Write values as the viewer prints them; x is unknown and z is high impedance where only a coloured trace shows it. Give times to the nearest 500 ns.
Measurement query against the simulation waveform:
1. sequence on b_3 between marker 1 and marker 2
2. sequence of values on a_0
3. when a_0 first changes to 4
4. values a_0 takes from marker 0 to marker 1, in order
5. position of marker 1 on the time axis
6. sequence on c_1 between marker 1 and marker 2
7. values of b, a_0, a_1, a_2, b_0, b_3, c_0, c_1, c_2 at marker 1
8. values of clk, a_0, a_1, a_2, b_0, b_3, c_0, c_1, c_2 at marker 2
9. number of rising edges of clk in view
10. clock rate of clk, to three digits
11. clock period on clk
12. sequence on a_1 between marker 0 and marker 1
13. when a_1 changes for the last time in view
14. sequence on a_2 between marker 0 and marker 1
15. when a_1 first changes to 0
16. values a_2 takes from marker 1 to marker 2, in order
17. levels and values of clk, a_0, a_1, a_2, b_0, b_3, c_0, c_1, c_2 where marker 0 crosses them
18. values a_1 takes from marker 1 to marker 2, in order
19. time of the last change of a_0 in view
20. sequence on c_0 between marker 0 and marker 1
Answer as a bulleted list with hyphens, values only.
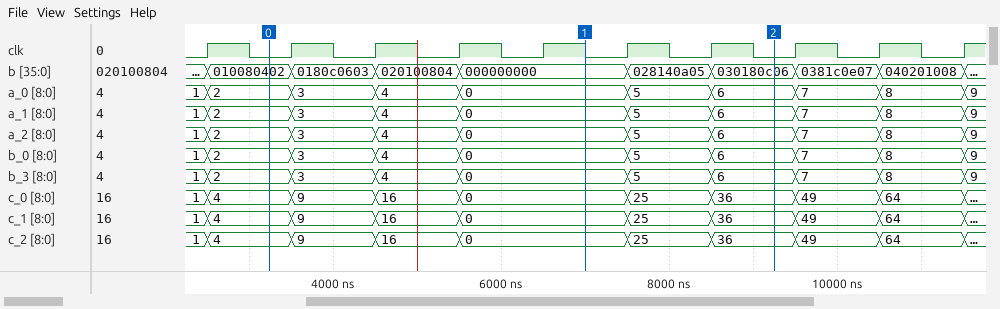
- 0, 5, 6
- 1, 2, 3, 4, 0, 5, 6, 7, 8, 9
- 4500 ns
- 2, 3, 4, 0
- 7000 ns
- 0, 25, 36
- b=000000000, a_0=0, a_1=0, a_2=0, b_0=0, b_3=0, c_0=0, c_1=0, c_2=0
- clk=0, a_0=6, a_1=6, a_2=6, b_0=6, b_3=6, c_0=36, c_1=36, c_2=36
- 10
- 1.00 MHz
- 1000 ns
- 2, 3, 4, 0
- 11500 ns
- 2, 3, 4, 0
- 5500 ns
- 0, 5, 6
- clk=0, a_0=2, a_1=2, a_2=2, b_0=2, b_3=2, c_0=4, c_1=4, c_2=4
- 0, 5, 6
- 11500 ns
- 4, 9, 16, 0
